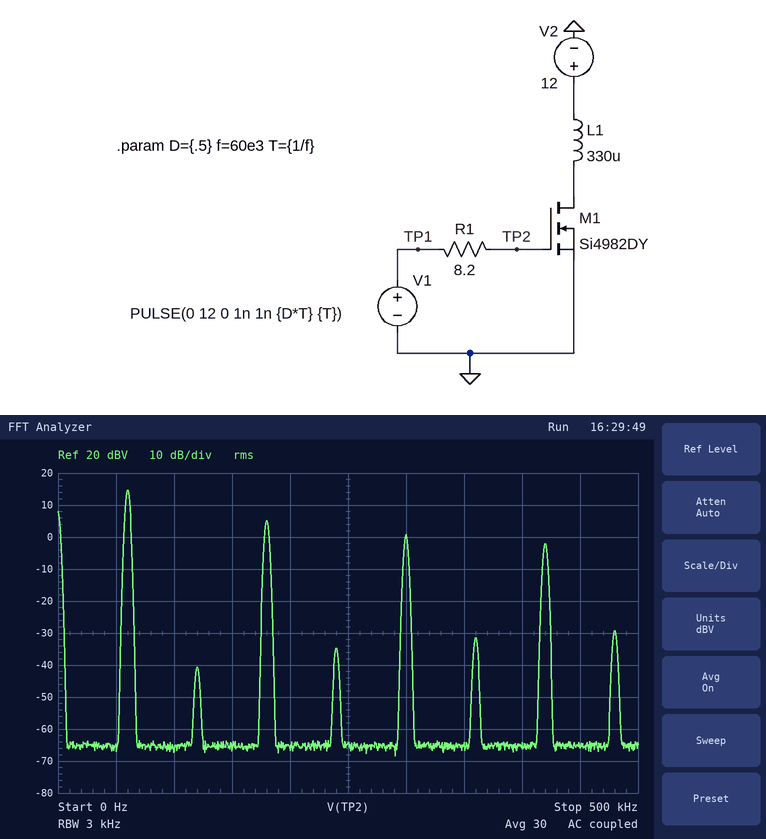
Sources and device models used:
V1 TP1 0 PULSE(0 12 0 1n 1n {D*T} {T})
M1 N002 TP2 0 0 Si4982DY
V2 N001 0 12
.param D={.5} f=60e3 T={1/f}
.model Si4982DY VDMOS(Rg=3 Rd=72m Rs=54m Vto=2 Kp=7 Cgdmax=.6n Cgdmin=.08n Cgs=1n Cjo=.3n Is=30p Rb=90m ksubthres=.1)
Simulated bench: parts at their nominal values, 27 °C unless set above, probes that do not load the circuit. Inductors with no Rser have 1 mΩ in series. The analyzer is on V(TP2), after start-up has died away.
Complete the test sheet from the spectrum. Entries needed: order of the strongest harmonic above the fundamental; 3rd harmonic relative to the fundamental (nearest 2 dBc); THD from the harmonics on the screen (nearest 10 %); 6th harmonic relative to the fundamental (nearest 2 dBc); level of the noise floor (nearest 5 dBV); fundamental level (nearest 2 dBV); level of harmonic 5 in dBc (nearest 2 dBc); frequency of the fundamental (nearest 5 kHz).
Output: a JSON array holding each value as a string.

["3", "-10 dBc", "40 %", "-46 dBc", "-65 dBV", "14 dBV", "-14 dBc", "60 kHz"]
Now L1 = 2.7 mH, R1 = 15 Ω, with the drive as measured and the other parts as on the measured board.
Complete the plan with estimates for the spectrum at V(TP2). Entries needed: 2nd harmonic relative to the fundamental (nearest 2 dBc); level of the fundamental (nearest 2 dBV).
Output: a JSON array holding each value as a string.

["-50 dBc", "14 dBV"]
